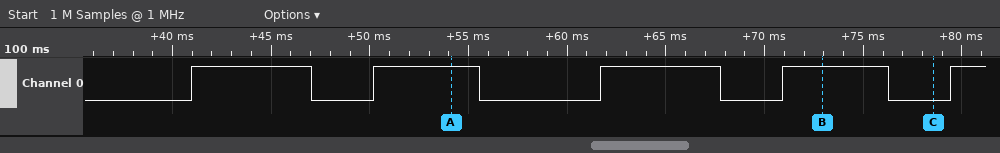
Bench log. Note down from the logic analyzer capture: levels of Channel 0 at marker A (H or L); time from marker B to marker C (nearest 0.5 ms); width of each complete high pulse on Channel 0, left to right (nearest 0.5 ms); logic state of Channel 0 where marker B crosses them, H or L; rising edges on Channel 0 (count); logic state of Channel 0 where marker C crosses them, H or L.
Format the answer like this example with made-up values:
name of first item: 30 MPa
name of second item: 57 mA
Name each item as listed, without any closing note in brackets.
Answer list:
levels of Channel 0 at marker A: Channel 0=H
time from marker B to marker C: 5.5 ms
width of each complete high pulse on Channel 0, left to right: 6 ms, 5.5 ms, 6 ms, 5.5 ms
logic state of Channel 0 where marker B crosses them, H or L: Channel 0=H
rising edges on Channel 0: 5
logic state of Channel 0 where marker C crosses them, H or L: Channel 0=L
